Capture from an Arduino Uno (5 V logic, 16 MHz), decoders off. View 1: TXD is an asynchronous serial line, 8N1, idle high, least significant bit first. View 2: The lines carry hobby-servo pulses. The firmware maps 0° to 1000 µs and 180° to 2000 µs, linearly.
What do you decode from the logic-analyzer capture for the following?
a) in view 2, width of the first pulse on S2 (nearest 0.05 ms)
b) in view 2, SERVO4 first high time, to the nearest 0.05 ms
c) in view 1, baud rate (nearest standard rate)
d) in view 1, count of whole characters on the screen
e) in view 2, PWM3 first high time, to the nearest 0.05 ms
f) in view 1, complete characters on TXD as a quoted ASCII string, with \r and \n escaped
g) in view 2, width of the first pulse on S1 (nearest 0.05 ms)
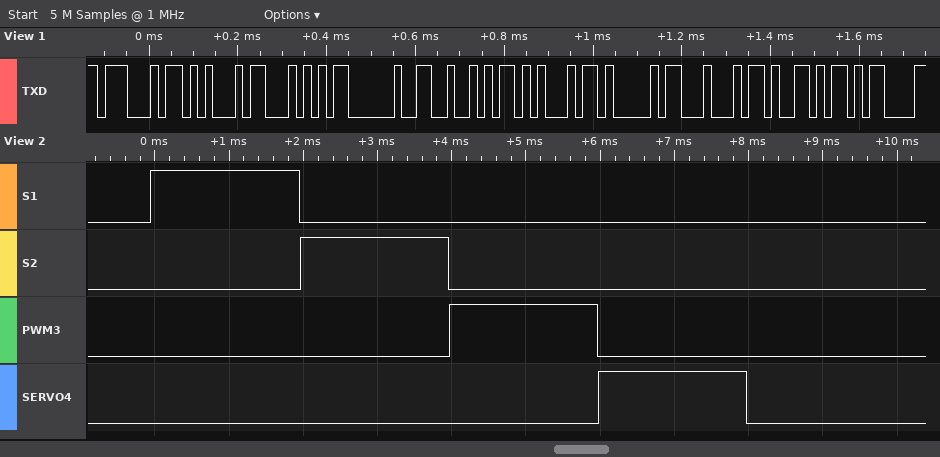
2.00 ms
2.00 ms
57600 baud
10
2.00 ms
"GET READY\r"
2.00 ms
